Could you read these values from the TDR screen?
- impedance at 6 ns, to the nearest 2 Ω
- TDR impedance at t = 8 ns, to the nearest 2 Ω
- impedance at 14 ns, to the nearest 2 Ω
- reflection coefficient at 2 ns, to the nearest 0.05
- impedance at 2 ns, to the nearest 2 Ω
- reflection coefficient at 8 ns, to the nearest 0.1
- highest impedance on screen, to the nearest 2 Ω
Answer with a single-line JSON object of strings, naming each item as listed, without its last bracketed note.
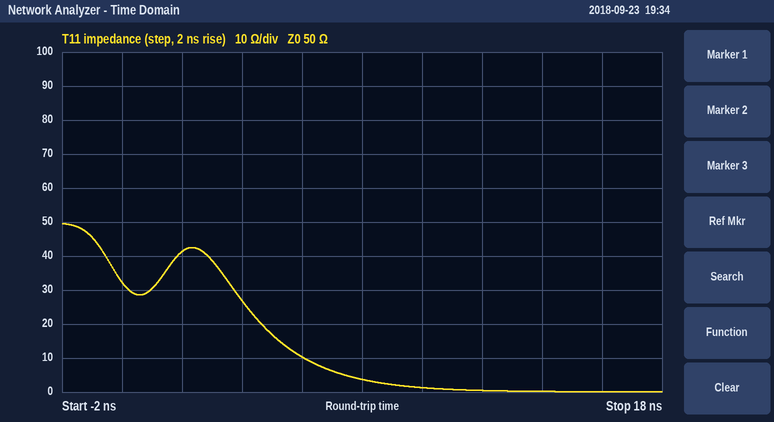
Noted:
{"impedance at 6 ns, to the nearest 2 Ω": "10 Ω", "TDR impedance at t = 8 ns, to the nearest 2 Ω": "4 Ω", "impedance at 14 ns, to the nearest 2 Ω": "0 Ω", "reflection coefficient at 2 ns, to the nearest 0.05": "-0.10", "impedance at 2 ns, to the nearest 2 Ω": "42 Ω", "reflection coefficient at 8 ns, to the nearest 0.1": "-0.9", "highest impedance on screen, to the nearest 2 Ω": "50 Ω"}
